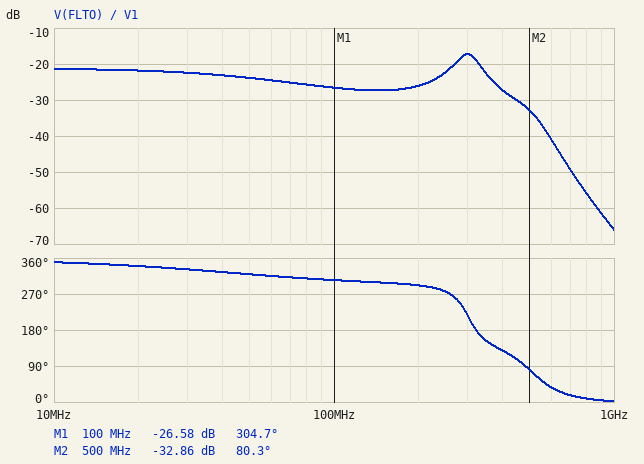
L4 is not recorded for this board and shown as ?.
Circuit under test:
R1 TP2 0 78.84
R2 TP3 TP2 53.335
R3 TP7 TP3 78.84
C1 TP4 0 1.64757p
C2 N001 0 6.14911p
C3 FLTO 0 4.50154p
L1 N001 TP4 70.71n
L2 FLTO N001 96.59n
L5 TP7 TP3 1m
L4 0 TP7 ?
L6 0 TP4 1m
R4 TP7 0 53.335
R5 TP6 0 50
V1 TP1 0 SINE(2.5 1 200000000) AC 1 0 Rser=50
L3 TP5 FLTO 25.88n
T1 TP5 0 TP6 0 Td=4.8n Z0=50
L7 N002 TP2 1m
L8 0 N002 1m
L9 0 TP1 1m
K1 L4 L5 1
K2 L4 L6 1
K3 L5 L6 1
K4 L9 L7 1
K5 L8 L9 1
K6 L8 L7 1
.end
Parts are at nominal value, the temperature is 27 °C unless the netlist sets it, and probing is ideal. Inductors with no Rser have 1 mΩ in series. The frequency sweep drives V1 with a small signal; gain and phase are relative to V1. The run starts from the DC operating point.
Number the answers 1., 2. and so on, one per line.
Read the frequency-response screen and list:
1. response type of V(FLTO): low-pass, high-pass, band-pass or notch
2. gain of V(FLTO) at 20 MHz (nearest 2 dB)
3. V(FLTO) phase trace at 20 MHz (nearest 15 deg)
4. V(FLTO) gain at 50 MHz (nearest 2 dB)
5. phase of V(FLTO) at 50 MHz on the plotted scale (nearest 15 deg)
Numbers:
1. low-pass
2. -22 dB
3. 345 deg
4. -24 dB
5. 315 deg
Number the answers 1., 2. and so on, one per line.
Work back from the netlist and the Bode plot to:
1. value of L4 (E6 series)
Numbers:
1. 3.3 mH
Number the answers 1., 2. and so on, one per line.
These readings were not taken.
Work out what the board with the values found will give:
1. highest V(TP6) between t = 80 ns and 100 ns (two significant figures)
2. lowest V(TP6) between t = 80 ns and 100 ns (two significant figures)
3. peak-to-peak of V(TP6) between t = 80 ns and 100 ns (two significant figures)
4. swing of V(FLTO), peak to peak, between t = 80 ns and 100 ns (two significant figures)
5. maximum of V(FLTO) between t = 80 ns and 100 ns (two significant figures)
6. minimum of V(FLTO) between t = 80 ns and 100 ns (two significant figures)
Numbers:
1. 42 mV
2. -42 mV
3. 83 mV
4. 99 mV
5. 50 mV
6. -50 mV
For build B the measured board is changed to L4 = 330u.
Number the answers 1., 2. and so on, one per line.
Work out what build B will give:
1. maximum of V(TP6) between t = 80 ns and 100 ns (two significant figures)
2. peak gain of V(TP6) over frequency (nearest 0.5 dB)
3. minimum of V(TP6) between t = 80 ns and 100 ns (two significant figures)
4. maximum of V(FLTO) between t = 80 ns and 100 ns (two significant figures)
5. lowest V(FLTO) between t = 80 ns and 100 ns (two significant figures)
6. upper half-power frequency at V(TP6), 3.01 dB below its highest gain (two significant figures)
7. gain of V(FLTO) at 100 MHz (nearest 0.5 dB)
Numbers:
1. 77 mV
2. -17.0 dB
3. -77 mV
4. 92 mV
5. -92 mV
6. 340 MHz
7. -21.5 dB
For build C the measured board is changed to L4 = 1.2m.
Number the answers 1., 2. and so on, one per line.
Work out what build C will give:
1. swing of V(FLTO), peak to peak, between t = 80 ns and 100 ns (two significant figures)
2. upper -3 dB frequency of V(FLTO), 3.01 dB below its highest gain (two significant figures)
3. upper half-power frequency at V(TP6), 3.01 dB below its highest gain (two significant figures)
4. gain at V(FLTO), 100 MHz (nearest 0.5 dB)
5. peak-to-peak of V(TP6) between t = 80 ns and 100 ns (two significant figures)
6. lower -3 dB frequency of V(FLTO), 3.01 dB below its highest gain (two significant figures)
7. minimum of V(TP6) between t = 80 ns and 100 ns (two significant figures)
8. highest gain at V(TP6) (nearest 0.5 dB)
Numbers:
1. 140 mV
2. 340 MHz
3. 330 MHz
4. -23.5 dB
5. 120 mV
6. 260 MHz
7. -59 mV
8. -18.0 dB
